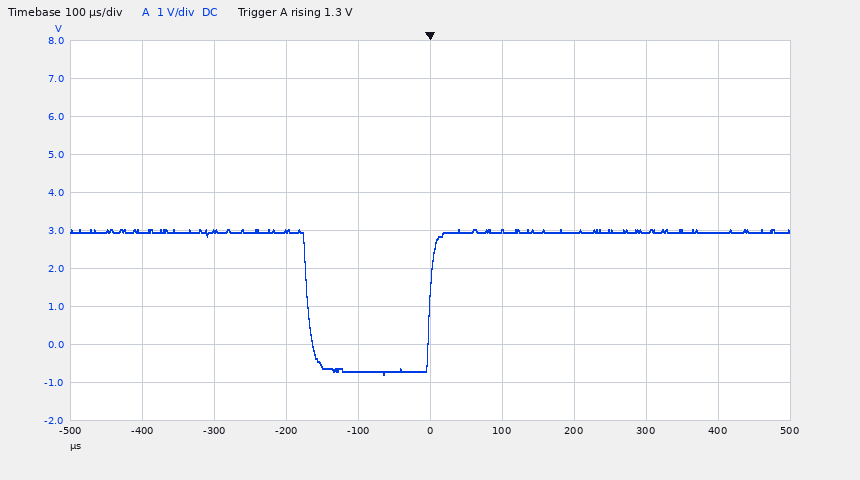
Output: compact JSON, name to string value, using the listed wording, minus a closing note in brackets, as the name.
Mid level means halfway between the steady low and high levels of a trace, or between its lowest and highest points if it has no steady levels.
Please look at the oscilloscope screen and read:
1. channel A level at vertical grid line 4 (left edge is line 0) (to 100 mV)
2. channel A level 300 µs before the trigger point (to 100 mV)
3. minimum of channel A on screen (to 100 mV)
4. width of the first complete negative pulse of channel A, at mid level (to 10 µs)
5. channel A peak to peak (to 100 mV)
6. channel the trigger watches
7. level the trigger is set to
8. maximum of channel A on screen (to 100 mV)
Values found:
{"channel A level at vertical grid line 4 (left edge is line 0)": "-700 mV", "channel A level 300 µs before the trigger point": "3.0 V", "minimum of channel A on screen": "-800 mV", "width of the first complete negative pulse of channel A, at mid level": "170 µs", "channel A peak to peak": "3.8 V", "channel the trigger watches": "channel A", "level the trigger is set to": "1.3 V", "maximum of channel A on screen": "3.0 V"}
